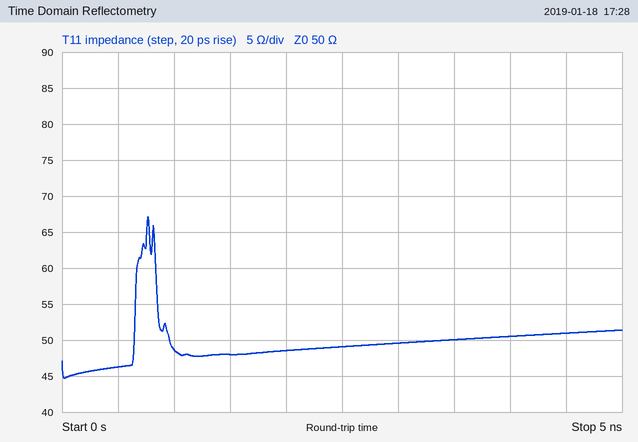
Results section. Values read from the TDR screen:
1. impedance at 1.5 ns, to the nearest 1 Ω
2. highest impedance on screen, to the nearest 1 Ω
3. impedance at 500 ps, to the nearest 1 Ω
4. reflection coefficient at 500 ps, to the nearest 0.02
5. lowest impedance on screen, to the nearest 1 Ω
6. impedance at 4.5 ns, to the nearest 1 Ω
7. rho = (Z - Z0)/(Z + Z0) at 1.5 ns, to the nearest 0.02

48 Ω
67 Ω
46 Ω
-0.04
45 Ω
51 Ω
-0.02
